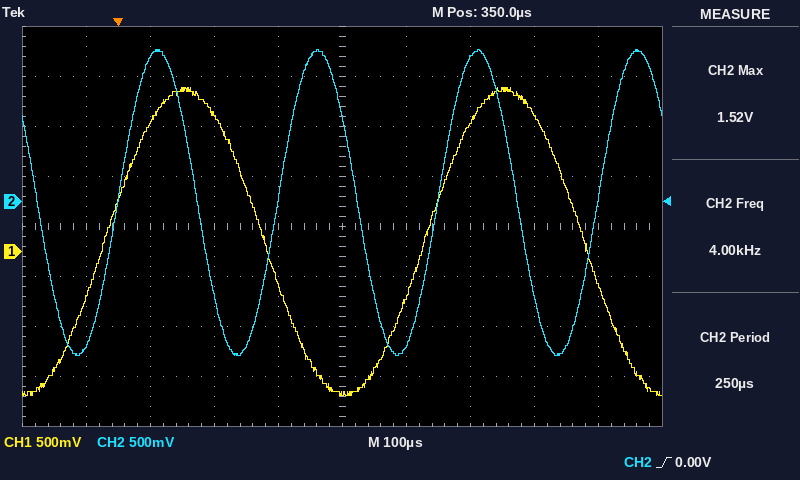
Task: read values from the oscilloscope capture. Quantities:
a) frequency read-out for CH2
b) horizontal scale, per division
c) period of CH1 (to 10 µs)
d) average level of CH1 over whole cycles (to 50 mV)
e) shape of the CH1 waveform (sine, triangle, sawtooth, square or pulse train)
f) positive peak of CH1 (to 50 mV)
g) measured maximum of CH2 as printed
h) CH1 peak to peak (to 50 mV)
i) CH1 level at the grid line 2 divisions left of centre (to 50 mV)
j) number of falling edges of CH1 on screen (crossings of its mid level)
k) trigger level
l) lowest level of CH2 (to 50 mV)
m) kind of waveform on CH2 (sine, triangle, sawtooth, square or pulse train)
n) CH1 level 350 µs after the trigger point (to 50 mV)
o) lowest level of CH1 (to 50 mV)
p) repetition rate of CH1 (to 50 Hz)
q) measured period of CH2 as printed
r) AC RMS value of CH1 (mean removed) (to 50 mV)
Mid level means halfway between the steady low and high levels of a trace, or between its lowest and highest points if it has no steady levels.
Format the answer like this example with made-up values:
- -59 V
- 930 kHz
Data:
- 4.00 kHz
- 100 µs
- 500 µs
- 100 mV
- sine
- 1.65 V
- 1.52 V
- 3.10 V
- 1.35 V
- 2
- 0.00 V
- -1.55 V
- sine
- -1.40 V
- -1.45 V
- 2.00 kHz
- 250 µs
- 1.10 V
